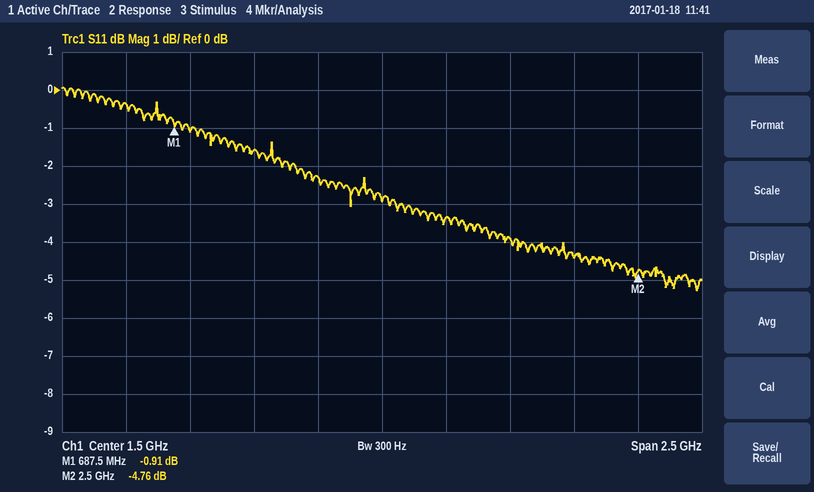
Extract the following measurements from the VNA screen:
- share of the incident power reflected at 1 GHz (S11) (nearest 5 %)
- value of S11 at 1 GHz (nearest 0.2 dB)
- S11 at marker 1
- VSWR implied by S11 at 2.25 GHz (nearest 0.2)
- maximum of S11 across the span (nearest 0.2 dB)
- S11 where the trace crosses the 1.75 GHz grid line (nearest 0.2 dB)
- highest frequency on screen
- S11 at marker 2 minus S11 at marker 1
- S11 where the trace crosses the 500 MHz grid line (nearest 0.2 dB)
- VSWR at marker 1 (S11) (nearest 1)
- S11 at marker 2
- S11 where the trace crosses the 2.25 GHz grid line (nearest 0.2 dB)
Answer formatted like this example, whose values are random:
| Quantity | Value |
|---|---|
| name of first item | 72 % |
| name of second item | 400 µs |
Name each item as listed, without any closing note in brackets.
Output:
| Quantity | Value |
|---|---|
| share of the incident power reflected at 1 GHz (S11) | 70 % |
| value of S11 at 1 GHz | -1.6 dB |
| S11 at marker 1 | -0.91 dB |
| VSWR implied by S11 at 2.25 GHz | 4.0 |
| maximum of S11 across the span | 0.0 dB |
| S11 where the trace crosses the 1.75 GHz grid line | -3.4 dB |
| highest frequency on screen | 2.75 GHz |
| S11 at marker 2 minus S11 at marker 1 | -3.85 dB |
| S11 where the trace crosses the 500 MHz grid line | -0.4 dB |
| VSWR at marker 1 (S11) | 19 |
| S11 at marker 2 | -4.76 dB |
| S11 where the trace crosses the 2.25 GHz grid line | -4.4 dB |
